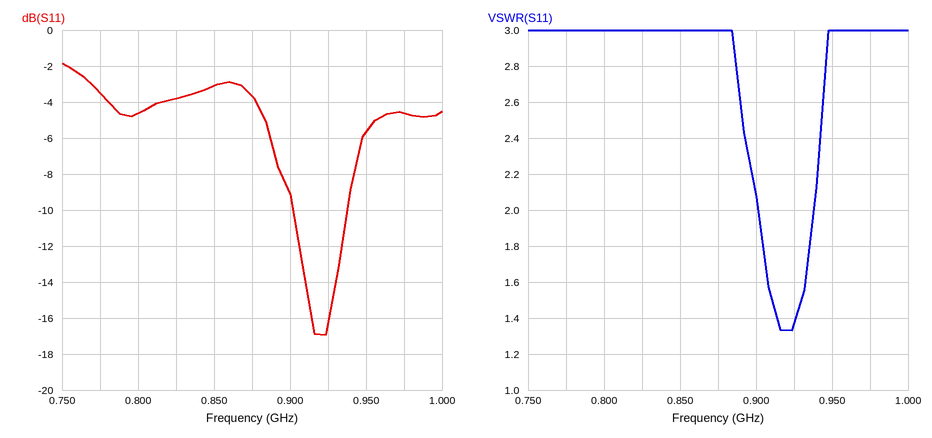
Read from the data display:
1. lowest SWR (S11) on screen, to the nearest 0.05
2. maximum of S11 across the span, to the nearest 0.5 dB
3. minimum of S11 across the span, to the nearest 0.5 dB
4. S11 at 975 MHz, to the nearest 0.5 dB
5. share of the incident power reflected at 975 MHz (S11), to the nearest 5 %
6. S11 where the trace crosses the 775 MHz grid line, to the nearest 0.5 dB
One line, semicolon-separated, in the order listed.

1.35; -2.0 dB; -17.0 dB; -4.5 dB; 35 %; -3.5 dB
